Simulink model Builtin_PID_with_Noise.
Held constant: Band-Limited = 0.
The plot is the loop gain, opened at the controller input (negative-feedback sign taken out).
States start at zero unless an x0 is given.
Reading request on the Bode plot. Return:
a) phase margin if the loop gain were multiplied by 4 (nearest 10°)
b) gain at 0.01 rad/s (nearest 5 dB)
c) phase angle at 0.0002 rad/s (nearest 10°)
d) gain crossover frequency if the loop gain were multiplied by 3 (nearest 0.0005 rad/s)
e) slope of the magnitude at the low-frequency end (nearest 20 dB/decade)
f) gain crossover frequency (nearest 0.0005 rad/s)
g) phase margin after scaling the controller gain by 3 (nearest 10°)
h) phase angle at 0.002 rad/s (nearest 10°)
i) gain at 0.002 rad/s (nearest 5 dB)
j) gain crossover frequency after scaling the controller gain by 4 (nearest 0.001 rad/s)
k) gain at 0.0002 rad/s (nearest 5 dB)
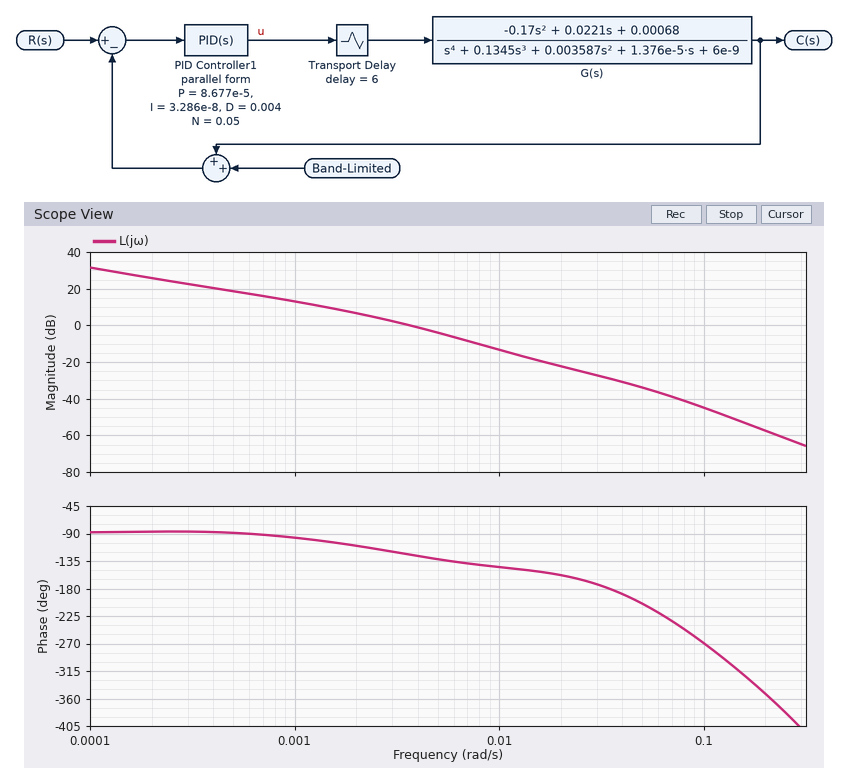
40°
-15 dB
-90°
0.0075 rad/s
-20 dB/decade
0.0035 rad/s
40°
-110°
5 dB
0.009 rad/s
25 dB
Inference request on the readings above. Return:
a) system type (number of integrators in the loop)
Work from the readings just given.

1
